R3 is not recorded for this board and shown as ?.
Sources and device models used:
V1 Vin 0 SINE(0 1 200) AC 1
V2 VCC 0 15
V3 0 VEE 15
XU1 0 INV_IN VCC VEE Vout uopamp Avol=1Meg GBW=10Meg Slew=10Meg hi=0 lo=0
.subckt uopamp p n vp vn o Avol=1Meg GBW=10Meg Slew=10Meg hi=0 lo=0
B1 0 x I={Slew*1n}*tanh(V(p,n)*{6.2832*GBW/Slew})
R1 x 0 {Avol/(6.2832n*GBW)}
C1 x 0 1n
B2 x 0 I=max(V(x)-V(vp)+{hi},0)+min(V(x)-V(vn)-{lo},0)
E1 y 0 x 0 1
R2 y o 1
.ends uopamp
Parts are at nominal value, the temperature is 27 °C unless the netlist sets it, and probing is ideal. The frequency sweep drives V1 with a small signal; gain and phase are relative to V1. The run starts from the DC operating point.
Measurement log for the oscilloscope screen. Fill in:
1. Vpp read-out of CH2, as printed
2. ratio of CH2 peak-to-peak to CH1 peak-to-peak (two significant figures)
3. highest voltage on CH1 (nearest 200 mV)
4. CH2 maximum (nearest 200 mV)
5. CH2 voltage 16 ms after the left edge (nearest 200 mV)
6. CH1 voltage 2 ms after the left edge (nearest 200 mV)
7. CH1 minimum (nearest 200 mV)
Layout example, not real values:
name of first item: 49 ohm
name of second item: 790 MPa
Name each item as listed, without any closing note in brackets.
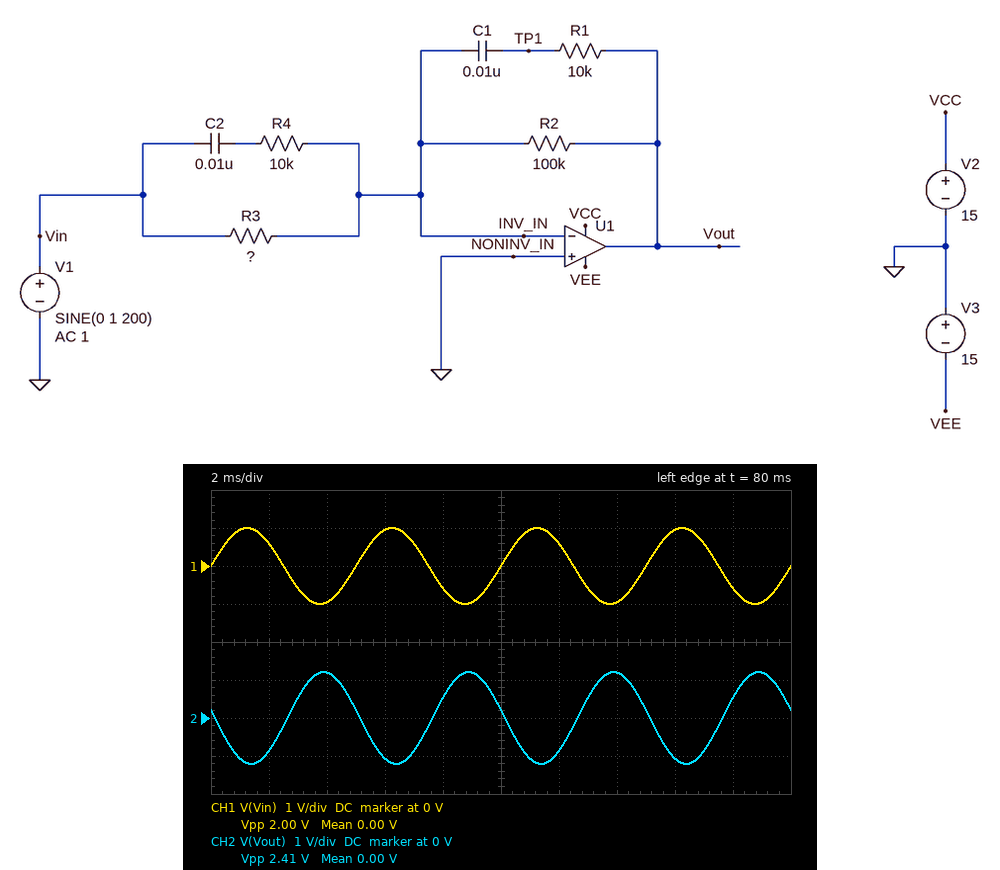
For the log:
Vpp read-out of CH2, as printed: 2.41 V
ratio of CH2 peak-to-peak to CH1 peak-to-peak: 1.2
highest voltage on CH1: 1.0 V
CH2 maximum: 1.2 V
CH2 voltage 16 ms after the left edge: -1.0 V
CH1 voltage 2 ms after the left edge: 600 mV
CH1 minimum: -1.0 V
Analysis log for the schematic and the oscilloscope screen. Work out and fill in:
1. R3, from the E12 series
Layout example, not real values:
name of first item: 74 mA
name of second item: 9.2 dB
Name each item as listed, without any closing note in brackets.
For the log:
R3, from the E12 series: 68 kΩ
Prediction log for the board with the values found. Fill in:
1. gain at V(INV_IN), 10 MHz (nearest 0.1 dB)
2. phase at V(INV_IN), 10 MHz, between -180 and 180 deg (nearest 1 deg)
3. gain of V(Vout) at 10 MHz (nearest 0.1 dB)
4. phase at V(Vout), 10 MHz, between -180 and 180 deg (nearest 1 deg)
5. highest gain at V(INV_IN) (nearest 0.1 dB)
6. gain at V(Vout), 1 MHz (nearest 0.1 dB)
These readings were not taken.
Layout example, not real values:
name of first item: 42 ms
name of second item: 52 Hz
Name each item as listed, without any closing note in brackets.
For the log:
gain at V(INV_IN), 10 MHz: -6.8 dB
phase at V(INV_IN), 10 MHz, between -180 and 180 deg: 26 deg
gain of V(Vout) at 10 MHz: -6.8 dB
phase at V(Vout), 10 MHz, between -180 and 180 deg: 116 deg
highest gain at V(INV_IN): -5.8 dB
gain at V(Vout), 1 MHz: 0.2 dB
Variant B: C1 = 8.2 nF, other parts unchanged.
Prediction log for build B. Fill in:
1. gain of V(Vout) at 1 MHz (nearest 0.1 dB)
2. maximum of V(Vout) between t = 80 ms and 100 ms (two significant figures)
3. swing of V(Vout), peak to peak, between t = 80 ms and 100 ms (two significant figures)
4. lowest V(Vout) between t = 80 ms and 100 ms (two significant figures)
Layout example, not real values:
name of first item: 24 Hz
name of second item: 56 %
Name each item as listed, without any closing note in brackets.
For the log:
gain of V(Vout) at 1 MHz: 0.2 dB
maximum of V(Vout) between t = 80 ms and 100 ms: 1.4 V
swing of V(Vout), peak to peak, between t = 80 ms and 100 ms: 2.7 V
lowest V(Vout) between t = 80 ms and 100 ms: -1.4 V
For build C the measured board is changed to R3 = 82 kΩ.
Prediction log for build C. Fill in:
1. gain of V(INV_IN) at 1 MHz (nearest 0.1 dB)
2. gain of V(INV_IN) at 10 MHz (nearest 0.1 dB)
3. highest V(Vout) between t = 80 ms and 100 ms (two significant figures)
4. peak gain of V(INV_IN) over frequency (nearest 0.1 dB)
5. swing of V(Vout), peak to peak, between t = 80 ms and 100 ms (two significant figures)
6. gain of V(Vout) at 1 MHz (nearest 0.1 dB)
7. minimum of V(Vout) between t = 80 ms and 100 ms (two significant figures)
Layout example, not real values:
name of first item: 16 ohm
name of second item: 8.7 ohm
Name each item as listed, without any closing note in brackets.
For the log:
gain of V(INV_IN) at 1 MHz: -20.0 dB
gain of V(INV_IN) at 10 MHz: -6.9 dB
highest V(Vout) between t = 80 ms and 100 ms: 1.1 V
peak gain of V(INV_IN) over frequency: -5.9 dB
swing of V(Vout), peak to peak, between t = 80 ms and 100 ms: 2.2 V
gain of V(Vout) at 1 MHz: 0 dB
minimum of V(Vout) between t = 80 ms and 100 ms: -1.1 V
